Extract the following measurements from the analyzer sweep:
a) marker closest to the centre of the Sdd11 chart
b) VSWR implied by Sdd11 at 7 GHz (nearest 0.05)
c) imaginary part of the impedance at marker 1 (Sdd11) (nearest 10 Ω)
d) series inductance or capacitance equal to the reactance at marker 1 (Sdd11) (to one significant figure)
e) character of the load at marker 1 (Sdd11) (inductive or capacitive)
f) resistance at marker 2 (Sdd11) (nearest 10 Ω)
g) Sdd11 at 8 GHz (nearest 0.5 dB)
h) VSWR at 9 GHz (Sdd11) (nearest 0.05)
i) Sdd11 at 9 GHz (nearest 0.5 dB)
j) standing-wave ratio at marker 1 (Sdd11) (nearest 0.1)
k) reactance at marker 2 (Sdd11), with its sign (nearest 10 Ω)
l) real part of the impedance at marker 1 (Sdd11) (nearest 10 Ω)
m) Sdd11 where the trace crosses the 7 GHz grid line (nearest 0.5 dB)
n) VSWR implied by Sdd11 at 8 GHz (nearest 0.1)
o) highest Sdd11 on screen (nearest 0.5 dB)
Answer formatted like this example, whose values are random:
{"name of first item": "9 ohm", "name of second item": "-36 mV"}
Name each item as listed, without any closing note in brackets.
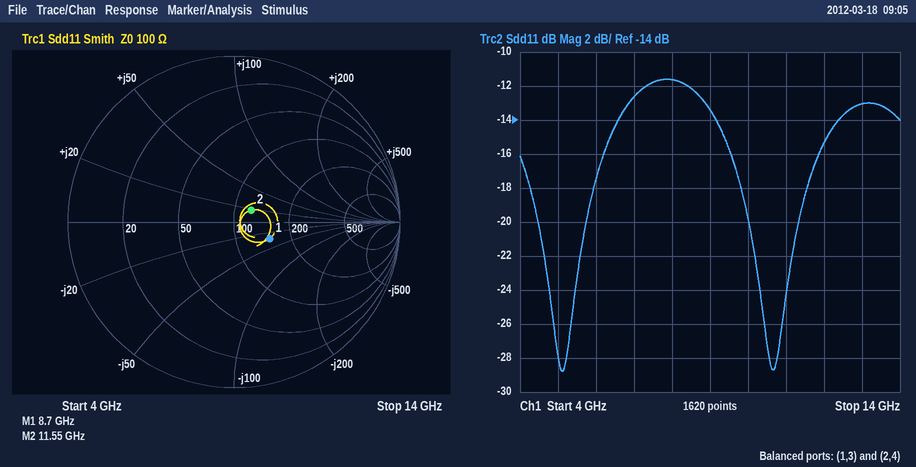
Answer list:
{"marker closest to the centre of the Sdd11 chart": "marker 2", "VSWR implied by Sdd11 at 7 GHz": "1.60", "imaginary part of the impedance at marker 1 (Sdd11)": "-30 Ω", "series inductance or capacitance equal to the reactance at marker 1 (Sdd11)": "600 fF", "character of the load at marker 1 (Sdd11)": "capacitive", "resistance at marker 2 (Sdd11)": "120 Ω", "Sdd11 at 8 GHz": "-11.5 dB", "VSWR at 9 GHz (Sdd11)": "1.55", "Sdd11 at 9 GHz": "-13.5 dB", "standing-wave ratio at marker 1 (Sdd11)": "1.6", "reactance at marker 2 (Sdd11), with its sign": "+20 Ω", "real part of the impedance at marker 1 (Sdd11)": "150 Ω", "Sdd11 where the trace crosses the 7 GHz grid line": "-12.5 dB", "VSWR implied by Sdd11 at 8 GHz": "1.7", "highest Sdd11 on screen": "-11.5 dB"}
